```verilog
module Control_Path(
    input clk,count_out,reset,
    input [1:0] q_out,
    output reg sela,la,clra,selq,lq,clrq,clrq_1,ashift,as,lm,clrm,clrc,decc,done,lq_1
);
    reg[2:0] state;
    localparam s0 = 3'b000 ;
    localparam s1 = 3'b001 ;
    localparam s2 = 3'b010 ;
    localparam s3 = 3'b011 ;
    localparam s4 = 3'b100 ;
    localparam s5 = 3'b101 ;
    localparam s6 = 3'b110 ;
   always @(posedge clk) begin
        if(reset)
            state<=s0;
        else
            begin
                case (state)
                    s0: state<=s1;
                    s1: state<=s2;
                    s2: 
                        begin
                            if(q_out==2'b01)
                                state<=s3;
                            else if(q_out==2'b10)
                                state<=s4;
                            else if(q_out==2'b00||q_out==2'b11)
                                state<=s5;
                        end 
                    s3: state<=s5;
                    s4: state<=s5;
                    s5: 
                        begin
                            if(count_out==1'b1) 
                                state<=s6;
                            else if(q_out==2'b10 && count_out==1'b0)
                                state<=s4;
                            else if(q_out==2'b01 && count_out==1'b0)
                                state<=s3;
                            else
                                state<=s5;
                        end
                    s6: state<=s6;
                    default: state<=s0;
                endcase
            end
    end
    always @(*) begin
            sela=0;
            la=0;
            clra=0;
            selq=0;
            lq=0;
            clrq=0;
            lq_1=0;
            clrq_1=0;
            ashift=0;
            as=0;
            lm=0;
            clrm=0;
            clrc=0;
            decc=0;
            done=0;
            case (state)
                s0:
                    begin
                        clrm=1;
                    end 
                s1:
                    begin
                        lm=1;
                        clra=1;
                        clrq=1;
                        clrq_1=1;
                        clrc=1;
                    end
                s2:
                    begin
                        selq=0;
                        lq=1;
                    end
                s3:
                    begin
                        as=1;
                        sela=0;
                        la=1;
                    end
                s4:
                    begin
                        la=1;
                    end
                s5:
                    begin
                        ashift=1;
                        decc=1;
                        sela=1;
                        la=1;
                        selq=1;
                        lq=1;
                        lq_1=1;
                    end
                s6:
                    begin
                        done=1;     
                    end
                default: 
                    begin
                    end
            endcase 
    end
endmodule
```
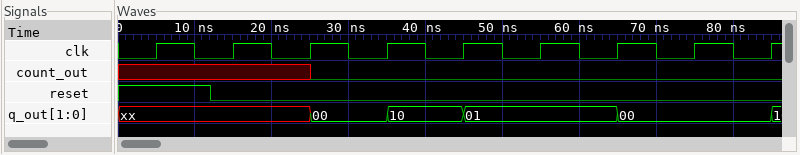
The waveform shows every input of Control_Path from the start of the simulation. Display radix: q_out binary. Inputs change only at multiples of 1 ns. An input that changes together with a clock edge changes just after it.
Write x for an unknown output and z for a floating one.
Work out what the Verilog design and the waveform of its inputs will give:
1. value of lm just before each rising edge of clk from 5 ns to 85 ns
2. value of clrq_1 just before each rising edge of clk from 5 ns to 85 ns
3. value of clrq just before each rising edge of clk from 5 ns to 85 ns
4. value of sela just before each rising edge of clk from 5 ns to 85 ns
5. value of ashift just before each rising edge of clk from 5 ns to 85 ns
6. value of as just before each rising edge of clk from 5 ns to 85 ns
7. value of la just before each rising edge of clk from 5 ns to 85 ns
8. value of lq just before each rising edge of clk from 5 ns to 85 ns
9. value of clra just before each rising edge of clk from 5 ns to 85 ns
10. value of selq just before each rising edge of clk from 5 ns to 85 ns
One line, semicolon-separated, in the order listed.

x 0 1 0 0 0 0 0 0; x 0 1 0 0 0 0 0 0; x 0 1 0 0 0 0 0 0; x 0 0 0 1 0 1 0 1; x 0 0 0 1 0 1 0 1; x 0 0 0 0 0 0 1 0; x 0 0 0 1 1 1 1 1; x 0 0 1 1 0 1 0 1; x 0 1 0 0 0 0 0 0; x 0 0 0 1 0 1 0 1
